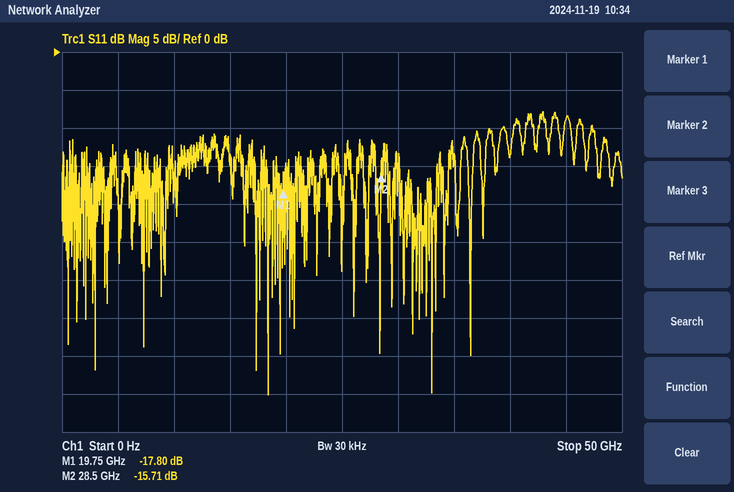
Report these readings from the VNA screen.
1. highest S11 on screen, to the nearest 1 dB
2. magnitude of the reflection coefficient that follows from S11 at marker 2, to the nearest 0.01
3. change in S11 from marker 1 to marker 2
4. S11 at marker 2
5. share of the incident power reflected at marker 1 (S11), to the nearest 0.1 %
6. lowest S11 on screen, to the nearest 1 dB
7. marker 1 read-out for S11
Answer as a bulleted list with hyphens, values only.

- -8 dB
- 0.16
- 2.09 dB
- -15.71 dB
- 1.7 %
- -45 dB
- -17.80 dB
